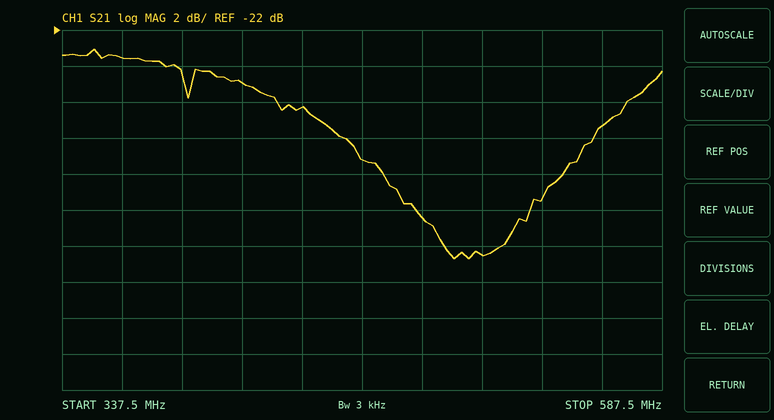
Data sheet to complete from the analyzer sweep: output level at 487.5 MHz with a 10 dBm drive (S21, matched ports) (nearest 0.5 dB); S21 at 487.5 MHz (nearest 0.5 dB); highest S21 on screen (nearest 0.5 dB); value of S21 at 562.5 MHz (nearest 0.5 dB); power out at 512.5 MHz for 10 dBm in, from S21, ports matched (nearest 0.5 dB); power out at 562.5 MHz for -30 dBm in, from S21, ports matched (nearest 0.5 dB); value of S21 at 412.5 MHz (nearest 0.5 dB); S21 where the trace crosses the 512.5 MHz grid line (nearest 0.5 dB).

-22.5 dBm
-32.5 dB
-23.0 dB
-27.5 dB
-24.5 dBm
-57.5 dBm
-25.0 dB
-34.5 dB
